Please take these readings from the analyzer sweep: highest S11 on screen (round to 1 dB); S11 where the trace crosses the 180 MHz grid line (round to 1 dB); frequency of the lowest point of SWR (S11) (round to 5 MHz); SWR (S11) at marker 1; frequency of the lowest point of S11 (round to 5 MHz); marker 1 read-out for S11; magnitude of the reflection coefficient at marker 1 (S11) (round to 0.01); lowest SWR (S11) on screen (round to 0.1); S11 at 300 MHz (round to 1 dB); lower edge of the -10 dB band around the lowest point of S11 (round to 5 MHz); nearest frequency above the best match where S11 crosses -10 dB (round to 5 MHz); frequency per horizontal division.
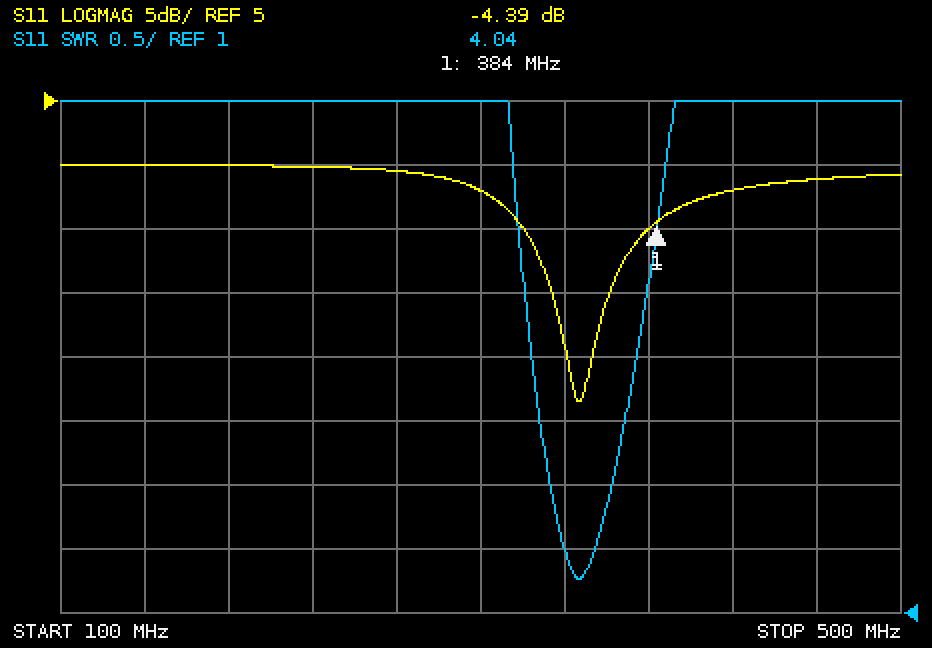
0 dB
0 dB
345 MHz
4.04
345 MHz
-4.39 dB
0.60
1.3
-2 dB
335 MHz
360 MHz
40 MHz
